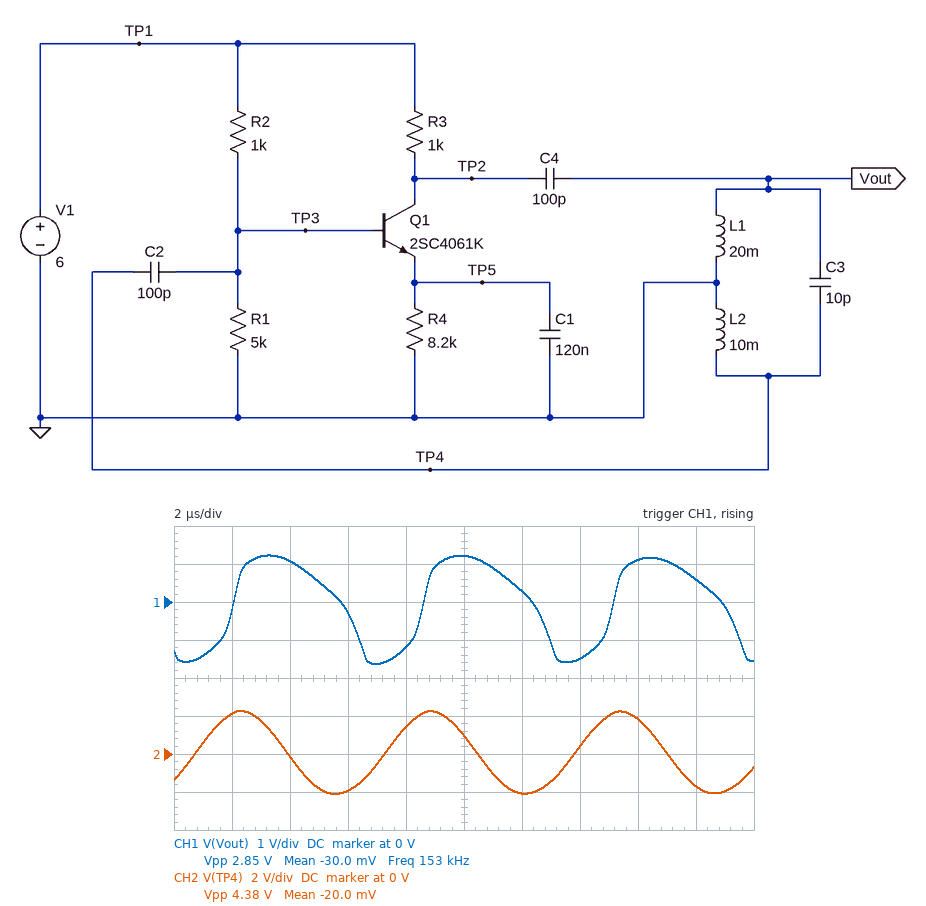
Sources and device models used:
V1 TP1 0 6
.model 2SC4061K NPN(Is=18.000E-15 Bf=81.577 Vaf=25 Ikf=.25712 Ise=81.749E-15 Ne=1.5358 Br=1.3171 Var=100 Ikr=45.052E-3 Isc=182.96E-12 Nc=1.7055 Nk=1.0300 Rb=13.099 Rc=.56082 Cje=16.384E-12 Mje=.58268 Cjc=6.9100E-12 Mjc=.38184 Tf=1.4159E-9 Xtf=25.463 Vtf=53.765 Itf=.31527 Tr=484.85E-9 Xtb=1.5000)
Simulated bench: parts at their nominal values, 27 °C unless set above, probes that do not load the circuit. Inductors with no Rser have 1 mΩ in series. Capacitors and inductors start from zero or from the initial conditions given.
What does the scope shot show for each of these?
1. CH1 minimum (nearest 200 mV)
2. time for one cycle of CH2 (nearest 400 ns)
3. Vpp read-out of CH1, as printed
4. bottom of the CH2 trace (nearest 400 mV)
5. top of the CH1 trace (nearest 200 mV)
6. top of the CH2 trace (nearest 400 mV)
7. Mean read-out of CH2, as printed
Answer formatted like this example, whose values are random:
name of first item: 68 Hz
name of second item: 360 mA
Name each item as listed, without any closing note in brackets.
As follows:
CH1 minimum: -1.6 V
time for one cycle of CH2: 6.4 µs
Vpp read-out of CH1, as printed: 2.85 V
bottom of the CH2 trace: -2.0 V
top of the CH1 trace: 1.2 V
top of the CH2 trace: 2.4 V
Mean read-out of CH2, as printed: -20.0 mV
